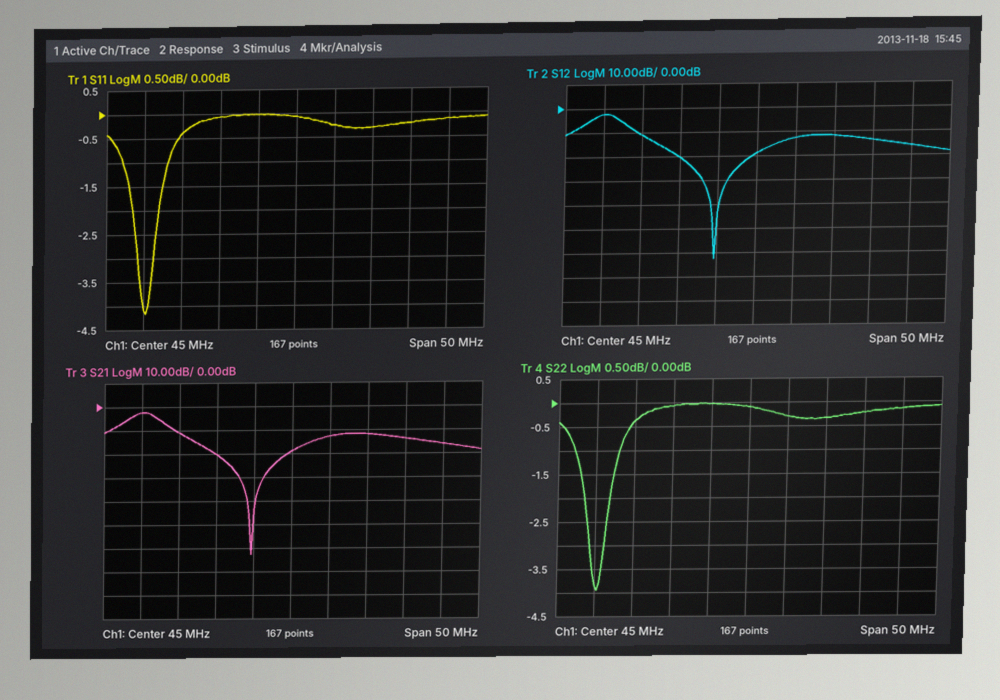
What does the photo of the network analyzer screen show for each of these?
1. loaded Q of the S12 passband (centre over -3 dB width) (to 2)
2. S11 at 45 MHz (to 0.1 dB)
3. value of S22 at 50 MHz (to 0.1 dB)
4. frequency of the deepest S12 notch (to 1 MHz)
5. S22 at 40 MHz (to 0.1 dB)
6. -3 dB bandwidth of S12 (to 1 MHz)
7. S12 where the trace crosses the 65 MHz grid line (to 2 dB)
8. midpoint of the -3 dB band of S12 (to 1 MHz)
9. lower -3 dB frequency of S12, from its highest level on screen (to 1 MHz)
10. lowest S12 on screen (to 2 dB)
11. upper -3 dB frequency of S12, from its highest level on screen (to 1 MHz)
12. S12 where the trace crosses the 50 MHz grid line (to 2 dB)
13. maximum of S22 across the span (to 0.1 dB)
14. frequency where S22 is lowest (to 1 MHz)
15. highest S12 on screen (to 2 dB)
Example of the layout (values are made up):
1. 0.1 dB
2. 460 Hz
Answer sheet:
1. 6
2. -0.1 dB
3. -0.3 dB
4. 40 MHz
5. 0.0 dB
6. 4 MHz
7. -16 dB
8. 25 MHz
9. 23 MHz
10. -62 dB
11. 27 MHz
12. -12 dB
13. 0.0 dB
14. 25 MHz
15. -2 dB
